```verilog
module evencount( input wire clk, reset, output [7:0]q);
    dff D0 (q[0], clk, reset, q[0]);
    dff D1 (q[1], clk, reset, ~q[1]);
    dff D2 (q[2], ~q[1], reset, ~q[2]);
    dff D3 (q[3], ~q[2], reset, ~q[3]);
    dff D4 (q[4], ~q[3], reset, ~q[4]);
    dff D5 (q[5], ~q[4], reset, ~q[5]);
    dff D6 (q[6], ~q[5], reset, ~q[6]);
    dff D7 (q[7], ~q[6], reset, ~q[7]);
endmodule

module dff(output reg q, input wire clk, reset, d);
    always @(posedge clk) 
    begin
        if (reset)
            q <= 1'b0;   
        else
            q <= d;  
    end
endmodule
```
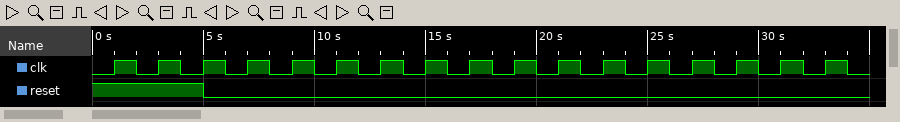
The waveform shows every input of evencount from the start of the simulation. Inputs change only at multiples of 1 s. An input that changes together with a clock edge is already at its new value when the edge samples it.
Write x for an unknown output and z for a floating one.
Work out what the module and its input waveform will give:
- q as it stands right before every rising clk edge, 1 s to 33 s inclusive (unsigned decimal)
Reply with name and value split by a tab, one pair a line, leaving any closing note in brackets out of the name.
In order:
q as it stands right before every rising clk edge, 1 s to 33 s inclusive	x, 0, 0, 2, 4, 6, 8, 10, 12, 14, 16, 18, 20, 22, 24, 26, 28
